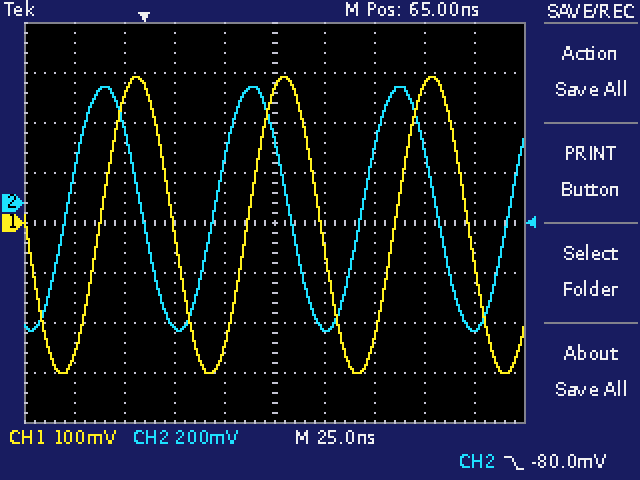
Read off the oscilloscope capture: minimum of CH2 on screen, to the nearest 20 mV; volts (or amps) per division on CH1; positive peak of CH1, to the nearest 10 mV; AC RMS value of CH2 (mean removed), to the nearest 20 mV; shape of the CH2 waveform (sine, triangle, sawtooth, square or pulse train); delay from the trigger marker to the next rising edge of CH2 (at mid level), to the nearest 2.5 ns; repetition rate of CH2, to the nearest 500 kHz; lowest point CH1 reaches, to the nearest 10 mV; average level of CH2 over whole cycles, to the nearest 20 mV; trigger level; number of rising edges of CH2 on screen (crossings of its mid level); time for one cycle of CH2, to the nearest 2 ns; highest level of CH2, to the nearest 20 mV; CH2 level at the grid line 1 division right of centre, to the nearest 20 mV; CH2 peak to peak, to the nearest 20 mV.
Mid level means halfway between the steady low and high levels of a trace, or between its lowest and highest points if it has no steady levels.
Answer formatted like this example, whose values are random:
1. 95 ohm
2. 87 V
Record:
1. -520 mV
2. 100 mV
3. 290 mV
4. 340 mV
5. sine
6. 35.0 ns
7. 13.5 MHz
8. -300 mV
9. -20 mV
10. -80.0 mV
11. 4
12. 74 ns
13. 460 mV
14. -500 mV
15. 980 mV
